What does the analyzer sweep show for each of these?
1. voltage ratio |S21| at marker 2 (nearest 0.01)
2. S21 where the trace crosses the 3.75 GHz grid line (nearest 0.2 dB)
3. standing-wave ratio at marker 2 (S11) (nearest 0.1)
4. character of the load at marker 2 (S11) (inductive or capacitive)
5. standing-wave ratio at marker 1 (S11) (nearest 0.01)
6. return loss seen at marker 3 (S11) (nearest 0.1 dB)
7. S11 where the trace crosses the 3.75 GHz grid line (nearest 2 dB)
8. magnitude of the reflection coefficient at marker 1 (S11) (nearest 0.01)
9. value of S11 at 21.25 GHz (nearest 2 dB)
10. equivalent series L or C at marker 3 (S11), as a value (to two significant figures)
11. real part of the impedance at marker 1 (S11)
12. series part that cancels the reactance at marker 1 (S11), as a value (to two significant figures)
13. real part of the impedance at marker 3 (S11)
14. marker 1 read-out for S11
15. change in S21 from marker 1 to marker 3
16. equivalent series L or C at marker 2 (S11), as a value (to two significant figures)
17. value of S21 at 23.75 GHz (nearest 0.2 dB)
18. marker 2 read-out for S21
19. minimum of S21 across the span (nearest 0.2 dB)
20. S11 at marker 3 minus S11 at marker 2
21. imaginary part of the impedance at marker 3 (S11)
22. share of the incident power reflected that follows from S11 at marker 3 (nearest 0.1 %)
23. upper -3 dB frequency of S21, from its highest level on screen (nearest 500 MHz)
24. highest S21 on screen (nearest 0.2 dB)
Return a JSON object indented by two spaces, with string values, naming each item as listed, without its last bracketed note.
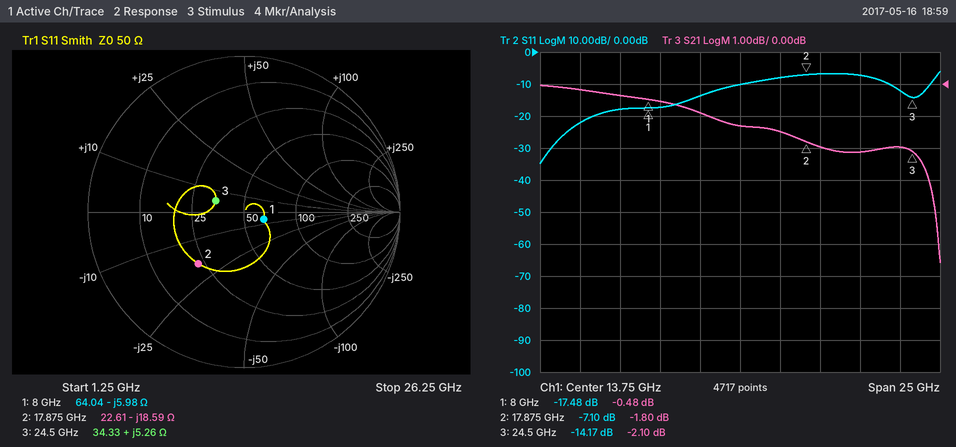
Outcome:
{
  "voltage ratio |S21| at marker 2": "0.81",
  "S21 where the trace crosses the 3.75 GHz grid line": "-0.2 dB",
  "standing-wave ratio at marker 2 (S11)": "2.6",
  "character of the load at marker 2 (S11)": "capacitive",
  "standing-wave ratio at marker 1 (S11)": "1.31",
  "return loss seen at marker 3 (S11)": "14.2 dB",
  "S11 where the trace crosses the 3.75 GHz grid line": "-22 dB",
  "magnitude of the reflection coefficient at marker 1 (S11)": "0.13",
  "value of S11 at 21.25 GHz": "-8 dB",
  "equivalent series L or C at marker 3 (S11), as a value": "34 pH",
  "real part of the impedance at marker 1": "64.04 Ω",
  "series part that cancels the reactance at marker 1 (S11), as a value": "120 pH",
  "real part of the impedance at marker 3": "34.33 Ω",
  "marker 1 read-out for S11": "-17.48 dB",
  "change in S21 from marker 1 to marker 3": "-1.62 dB",
  "equivalent series L or C at marker 2 (S11), as a value": "480 fF",
  "value of S21 at 23.75 GHz": "-2.0 dB",
  "marker 2 read-out for S21": "-1.80 dB",
  "minimum of S21 across the span": "-5.6 dB",
  "S11 at marker 3 minus S11 at marker 2": "-7.07 dB",
  "imaginary part of the impedance at marker 3": "+5.26 Ω",
  "share of the incident power reflected that follows from S11 at marker 3": "3.8 %",
  "upper -3 dB frequency of S21, from its highest level on screen": "25.5 GHz",
  "highest S21 on screen": "0.0 dB"
}
